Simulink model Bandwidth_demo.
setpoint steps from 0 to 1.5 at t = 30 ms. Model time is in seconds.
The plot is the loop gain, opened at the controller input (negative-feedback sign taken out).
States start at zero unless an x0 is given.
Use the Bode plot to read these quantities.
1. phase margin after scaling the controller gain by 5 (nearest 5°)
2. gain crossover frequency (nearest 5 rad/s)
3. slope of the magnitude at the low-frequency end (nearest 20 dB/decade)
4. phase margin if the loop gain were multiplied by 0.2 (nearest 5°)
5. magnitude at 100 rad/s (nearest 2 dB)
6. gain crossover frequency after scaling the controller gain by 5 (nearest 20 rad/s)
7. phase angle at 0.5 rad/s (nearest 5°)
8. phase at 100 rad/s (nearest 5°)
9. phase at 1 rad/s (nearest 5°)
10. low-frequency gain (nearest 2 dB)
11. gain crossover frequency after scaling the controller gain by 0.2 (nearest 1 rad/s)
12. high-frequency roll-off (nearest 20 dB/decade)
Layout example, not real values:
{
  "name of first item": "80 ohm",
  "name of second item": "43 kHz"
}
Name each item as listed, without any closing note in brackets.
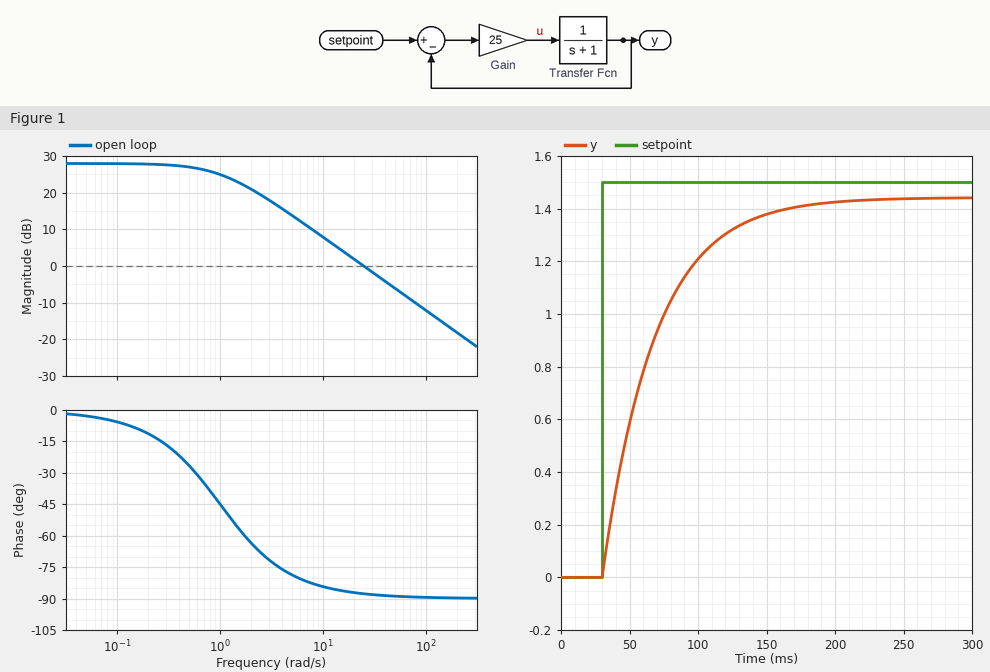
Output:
{
  "phase margin after scaling the controller gain by 5": "90°",
  "gain crossover frequency": "25 rad/s",
  "slope of the magnitude at the low-frequency end": "0 dB/decade",
  "phase margin if the loop gain were multiplied by 0.2": "100°",
  "magnitude at 100 rad/s": "-12 dB",
  "gain crossover frequency after scaling the controller gain by 5": "120 rad/s",
  "phase angle at 0.5 rad/s": "-25°",
  "phase at 100 rad/s": "-90°",
  "phase at 1 rad/s": "-45°",
  "low-frequency gain": "28 dB",
  "gain crossover frequency after scaling the controller gain by 0.2": "5 rad/s",
  "high-frequency roll-off": "-20 dB/decade"
}
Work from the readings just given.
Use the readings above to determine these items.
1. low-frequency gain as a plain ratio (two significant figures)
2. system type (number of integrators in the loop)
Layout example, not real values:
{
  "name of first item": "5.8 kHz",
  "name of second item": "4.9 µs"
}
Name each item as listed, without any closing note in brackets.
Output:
{
  "low-frequency gain as a plain ratio": "25",
  "system type": "0"
}
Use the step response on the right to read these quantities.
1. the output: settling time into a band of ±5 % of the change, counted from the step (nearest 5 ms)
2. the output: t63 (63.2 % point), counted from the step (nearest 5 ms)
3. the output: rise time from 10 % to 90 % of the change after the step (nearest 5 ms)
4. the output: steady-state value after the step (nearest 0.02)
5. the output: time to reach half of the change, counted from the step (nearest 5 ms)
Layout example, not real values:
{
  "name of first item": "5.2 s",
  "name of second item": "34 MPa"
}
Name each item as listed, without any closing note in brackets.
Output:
{
  "the output: settling time into a band of ±5 % of the change, counted from the step": "115 ms",
  "the output: t63 (63.2 % point), counted from the step": "40 ms",
  "the output: rise time from 10 % to 90 % of the change after the step": "85 ms",
  "the output: steady-state value after the step": "1.44",
  "the output: time to reach half of the change, counted from the step": "25 ms"
}
